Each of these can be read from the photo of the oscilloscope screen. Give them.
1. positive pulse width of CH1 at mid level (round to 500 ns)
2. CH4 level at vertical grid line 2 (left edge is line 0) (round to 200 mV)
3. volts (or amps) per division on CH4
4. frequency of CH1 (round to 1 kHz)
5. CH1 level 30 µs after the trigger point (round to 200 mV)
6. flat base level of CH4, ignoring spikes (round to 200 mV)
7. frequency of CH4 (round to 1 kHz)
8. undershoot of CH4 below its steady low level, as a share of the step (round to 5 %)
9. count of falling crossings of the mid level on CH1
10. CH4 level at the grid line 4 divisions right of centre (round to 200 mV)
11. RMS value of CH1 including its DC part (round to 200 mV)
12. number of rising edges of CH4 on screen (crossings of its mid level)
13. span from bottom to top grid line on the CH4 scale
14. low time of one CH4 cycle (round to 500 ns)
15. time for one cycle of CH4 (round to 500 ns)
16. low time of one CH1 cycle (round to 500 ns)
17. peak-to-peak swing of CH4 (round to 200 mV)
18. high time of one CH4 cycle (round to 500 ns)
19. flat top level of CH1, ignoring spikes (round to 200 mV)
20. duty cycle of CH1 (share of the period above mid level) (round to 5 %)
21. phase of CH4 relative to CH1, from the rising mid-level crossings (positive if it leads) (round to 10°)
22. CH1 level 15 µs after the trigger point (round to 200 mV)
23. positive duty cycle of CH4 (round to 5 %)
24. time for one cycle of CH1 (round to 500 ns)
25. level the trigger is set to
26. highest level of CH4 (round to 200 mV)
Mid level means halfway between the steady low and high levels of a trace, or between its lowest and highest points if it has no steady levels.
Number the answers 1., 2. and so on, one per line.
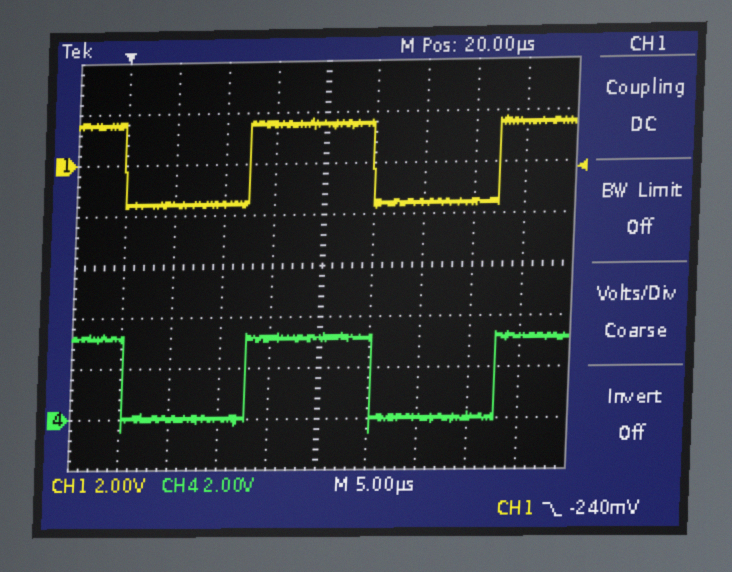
1. 12.5 µs
2. 0.0 V
3. 2 V
4. 40 kHz
5. -1.6 V
6. 0.0 V
7. 40 kHz
8. 20 %
9. 2
10. 3.2 V
11. 1.6 V
12. 2
13. 16 V
14. 12.5 µs
15. 25.0 µs
16. 12.5 µs
17. 4.0 V
18. 12.5 µs
19. 1.6 V
20. 50 %
21. 0°
22. 1.6 V
23. 50 %
24. 25.0 µs
25. -240 mV
26. 3.4 V
